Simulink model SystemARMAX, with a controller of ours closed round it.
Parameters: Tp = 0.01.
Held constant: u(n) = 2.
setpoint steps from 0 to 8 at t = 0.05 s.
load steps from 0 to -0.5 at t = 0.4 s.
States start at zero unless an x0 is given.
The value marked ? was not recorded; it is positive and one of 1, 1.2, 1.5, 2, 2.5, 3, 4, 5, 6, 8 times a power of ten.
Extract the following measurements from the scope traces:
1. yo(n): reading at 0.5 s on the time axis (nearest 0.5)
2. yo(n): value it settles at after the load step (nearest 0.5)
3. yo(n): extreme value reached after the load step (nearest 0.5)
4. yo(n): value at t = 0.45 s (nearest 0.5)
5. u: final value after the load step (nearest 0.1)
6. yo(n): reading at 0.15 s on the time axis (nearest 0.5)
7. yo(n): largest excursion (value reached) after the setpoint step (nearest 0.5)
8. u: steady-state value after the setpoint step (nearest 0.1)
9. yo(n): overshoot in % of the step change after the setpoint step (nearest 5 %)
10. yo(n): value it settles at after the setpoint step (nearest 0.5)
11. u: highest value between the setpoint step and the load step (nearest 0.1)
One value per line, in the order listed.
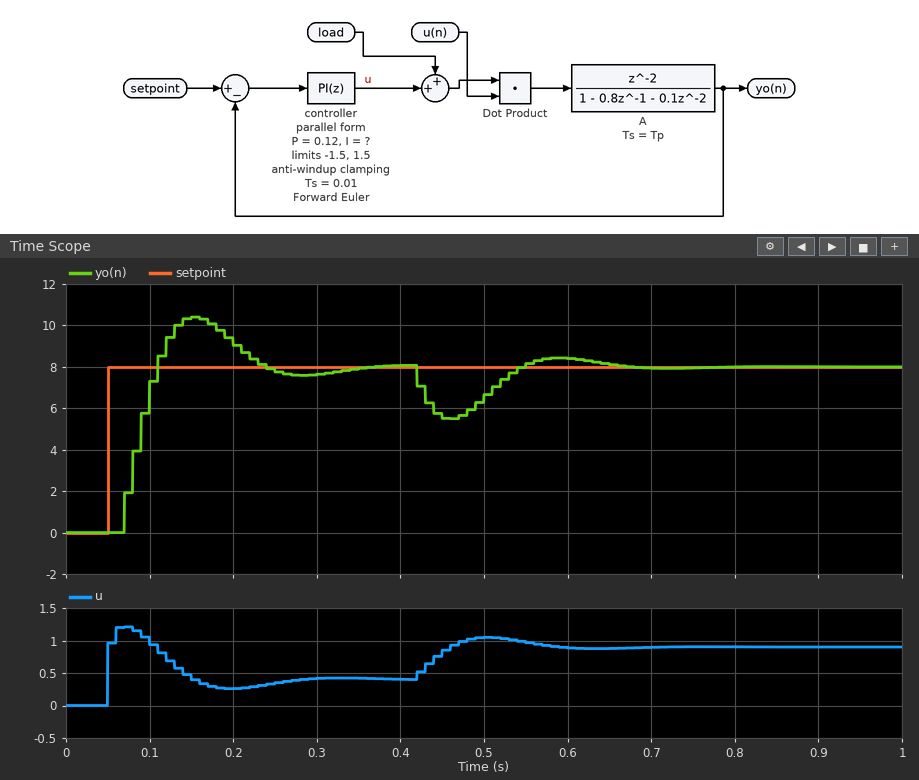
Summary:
6.5
8.0
5.5
5.5
0.9
10.5
10.5
0.4
30 %
8.0
1.2
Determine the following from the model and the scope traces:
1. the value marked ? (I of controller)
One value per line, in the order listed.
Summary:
3
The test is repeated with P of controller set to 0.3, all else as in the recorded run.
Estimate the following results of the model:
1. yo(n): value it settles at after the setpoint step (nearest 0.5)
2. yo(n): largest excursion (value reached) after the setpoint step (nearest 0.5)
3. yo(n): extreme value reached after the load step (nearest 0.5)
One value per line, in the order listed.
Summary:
8.0
8.5
6.0
